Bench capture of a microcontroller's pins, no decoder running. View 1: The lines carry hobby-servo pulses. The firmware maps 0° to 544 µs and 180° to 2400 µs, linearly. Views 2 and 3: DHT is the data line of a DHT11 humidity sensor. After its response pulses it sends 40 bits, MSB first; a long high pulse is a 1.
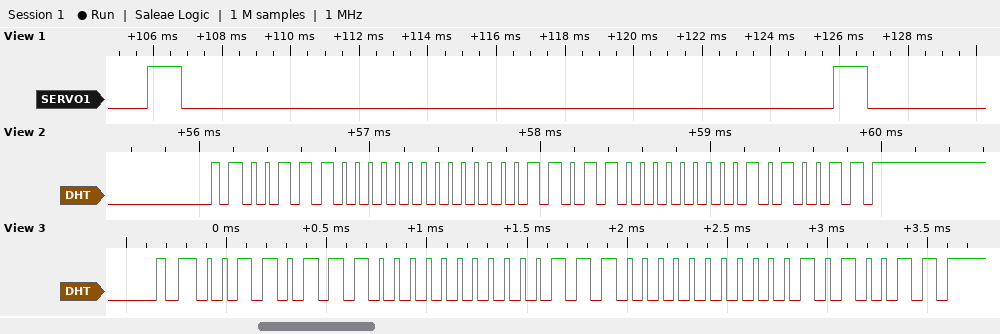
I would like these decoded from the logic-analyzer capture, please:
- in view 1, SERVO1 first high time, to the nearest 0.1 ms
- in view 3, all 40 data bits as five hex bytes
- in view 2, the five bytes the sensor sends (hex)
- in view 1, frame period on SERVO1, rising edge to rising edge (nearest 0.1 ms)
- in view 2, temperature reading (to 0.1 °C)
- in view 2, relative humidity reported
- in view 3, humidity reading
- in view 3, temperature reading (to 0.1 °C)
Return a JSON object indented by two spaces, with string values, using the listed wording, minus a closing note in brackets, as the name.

{
  "in view 1, SERVO1 first high time, to the nearest 0.1 ms": "1.0 ms",
  "in view 3, all 40 data bits as five hex bytes": "37 00 1C 00 53",
  "in view 2, the five bytes the sensor sends": "38 00 1B 00 53",
  "in view 1, frame period on SERVO1, rising edge to rising edge": "20.0 ms",
  "in view 2, temperature reading": "27.0 °C",
  "in view 2, relative humidity reported": "56 %",
  "in view 3, humidity reading": "55 %",
  "in view 3, temperature reading": "28.0 °C"
}
